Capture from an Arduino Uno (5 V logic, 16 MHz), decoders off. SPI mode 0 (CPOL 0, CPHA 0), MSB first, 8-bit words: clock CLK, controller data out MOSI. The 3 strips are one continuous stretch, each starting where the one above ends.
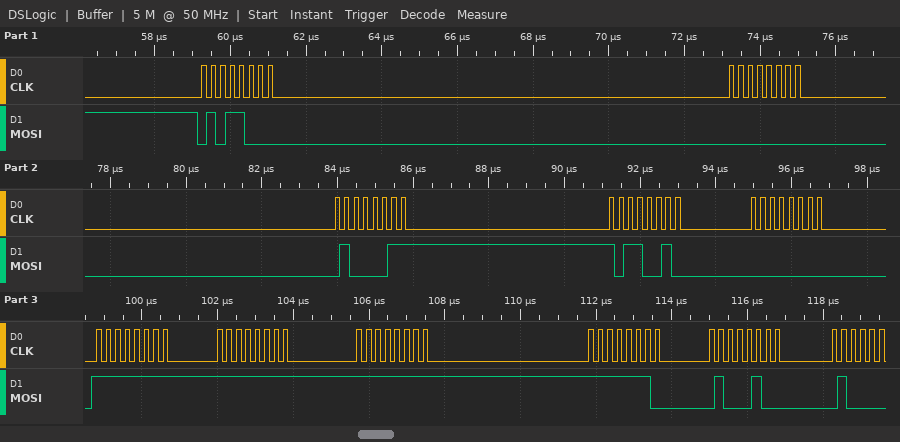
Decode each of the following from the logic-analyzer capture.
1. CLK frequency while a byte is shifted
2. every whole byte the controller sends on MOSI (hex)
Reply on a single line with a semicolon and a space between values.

4 MHz; 0x58 0x00 0x43 0xB2 0x00 0xFF 0xFF 0xFF 0xFE 0x44
